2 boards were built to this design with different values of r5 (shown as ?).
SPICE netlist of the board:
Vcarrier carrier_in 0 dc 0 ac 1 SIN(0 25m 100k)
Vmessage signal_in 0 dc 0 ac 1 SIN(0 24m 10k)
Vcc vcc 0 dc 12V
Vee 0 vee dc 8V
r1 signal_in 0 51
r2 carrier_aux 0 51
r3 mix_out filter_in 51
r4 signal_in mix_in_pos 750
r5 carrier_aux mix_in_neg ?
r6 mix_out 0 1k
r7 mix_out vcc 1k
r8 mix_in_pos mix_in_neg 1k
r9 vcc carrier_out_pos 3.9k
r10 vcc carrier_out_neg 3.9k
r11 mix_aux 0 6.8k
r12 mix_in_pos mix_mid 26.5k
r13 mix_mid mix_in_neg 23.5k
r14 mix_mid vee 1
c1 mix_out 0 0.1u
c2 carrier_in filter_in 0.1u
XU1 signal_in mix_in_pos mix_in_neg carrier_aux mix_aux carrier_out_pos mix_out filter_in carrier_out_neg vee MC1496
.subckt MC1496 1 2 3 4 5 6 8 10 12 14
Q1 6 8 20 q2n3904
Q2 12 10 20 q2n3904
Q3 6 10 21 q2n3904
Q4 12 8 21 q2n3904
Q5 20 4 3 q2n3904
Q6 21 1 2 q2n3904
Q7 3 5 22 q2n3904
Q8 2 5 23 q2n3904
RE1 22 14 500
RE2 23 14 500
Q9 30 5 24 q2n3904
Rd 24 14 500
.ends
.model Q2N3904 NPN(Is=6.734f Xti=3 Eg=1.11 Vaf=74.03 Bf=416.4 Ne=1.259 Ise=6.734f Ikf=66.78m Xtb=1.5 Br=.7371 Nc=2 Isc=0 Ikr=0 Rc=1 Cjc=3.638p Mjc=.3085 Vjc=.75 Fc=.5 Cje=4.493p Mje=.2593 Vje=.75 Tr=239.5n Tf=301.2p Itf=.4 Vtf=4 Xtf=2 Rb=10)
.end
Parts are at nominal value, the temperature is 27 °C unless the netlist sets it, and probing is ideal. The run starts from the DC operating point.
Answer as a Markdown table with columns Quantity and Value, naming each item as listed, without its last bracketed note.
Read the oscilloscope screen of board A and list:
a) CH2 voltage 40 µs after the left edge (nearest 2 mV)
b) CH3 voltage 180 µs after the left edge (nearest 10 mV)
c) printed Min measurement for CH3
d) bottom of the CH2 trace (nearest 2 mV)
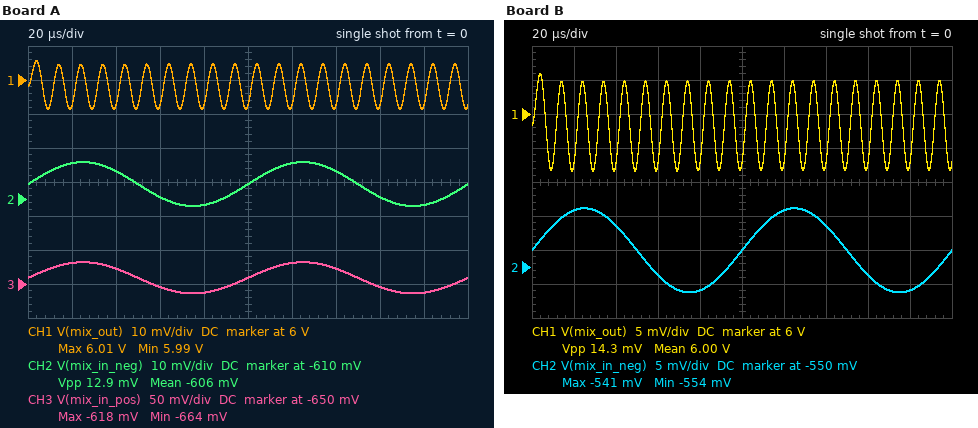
| Quantity | Value |
|---|---|
| CH2 voltage 40 µs after the left edge | -602 mV |
| CH3 voltage 180 µs after the left edge | -660 mV |
| printed Min measurement for CH3 | -664 mV |
| bottom of the CH2 trace | -612 mV |
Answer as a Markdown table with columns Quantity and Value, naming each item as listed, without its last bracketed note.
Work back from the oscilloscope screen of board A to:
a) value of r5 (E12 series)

| Quantity | Value |
|---|---|
| value of r5 | 390 Ω |
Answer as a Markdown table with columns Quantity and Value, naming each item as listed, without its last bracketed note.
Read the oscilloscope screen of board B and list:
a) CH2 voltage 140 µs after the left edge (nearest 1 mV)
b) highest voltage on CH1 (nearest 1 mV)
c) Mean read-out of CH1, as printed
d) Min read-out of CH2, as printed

| Quantity | Value |
|---|---|
| CH2 voltage 140 µs after the left edge | -544 mV |
| highest voltage on CH1 | 6.006 V |
| Mean read-out of CH1, as printed | 6.00 V |
| Min read-out of CH2, as printed | -554 mV |
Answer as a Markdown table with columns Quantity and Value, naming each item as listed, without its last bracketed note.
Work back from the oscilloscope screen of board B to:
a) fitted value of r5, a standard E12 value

| Quantity | Value |
|---|---|
| fitted value of r5, a standard E12 value | 330 Ω |
